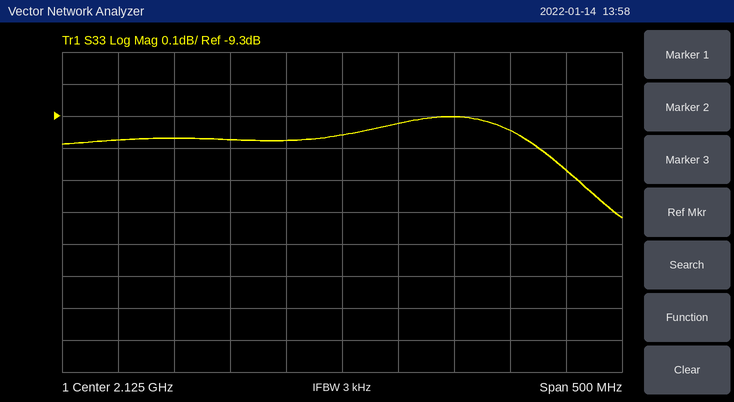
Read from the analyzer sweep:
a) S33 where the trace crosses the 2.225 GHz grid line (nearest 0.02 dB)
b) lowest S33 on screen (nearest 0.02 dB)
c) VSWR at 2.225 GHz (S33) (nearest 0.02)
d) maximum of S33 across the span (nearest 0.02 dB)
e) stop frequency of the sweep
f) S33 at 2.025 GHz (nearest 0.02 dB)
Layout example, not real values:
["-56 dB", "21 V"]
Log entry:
["-9.30 dB", "-9.62 dB", "2.04", "-9.30 dB", "2.375 GHz", "-9.38 dB"]
